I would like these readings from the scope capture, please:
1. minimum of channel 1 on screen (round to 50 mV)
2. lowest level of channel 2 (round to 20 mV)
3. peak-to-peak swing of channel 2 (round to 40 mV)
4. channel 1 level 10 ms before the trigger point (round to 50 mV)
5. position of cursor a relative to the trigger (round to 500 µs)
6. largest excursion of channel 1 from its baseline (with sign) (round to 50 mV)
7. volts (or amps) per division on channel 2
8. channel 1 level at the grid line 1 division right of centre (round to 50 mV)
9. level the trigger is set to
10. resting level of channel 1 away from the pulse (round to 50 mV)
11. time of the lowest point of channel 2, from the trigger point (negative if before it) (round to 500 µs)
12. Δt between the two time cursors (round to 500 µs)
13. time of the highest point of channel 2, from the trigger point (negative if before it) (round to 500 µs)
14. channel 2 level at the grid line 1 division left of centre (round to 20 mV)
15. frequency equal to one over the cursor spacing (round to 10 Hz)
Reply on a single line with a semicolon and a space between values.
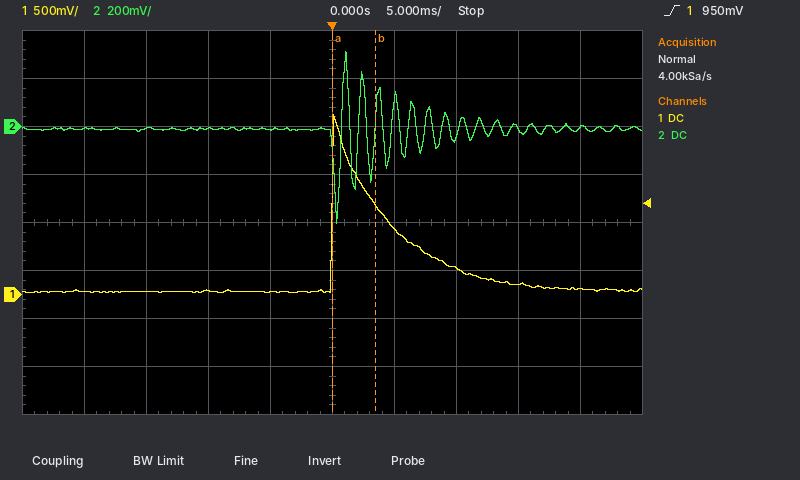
0 mV; -400 mV; 720 mV; 50 mV; 0.0 ms; +1.85 V; 200 mV; 700 mV; 950 mV; 50 mV; +500 µs; 3.5 ms; +1.0 ms; -20 mV; 290 Hz
